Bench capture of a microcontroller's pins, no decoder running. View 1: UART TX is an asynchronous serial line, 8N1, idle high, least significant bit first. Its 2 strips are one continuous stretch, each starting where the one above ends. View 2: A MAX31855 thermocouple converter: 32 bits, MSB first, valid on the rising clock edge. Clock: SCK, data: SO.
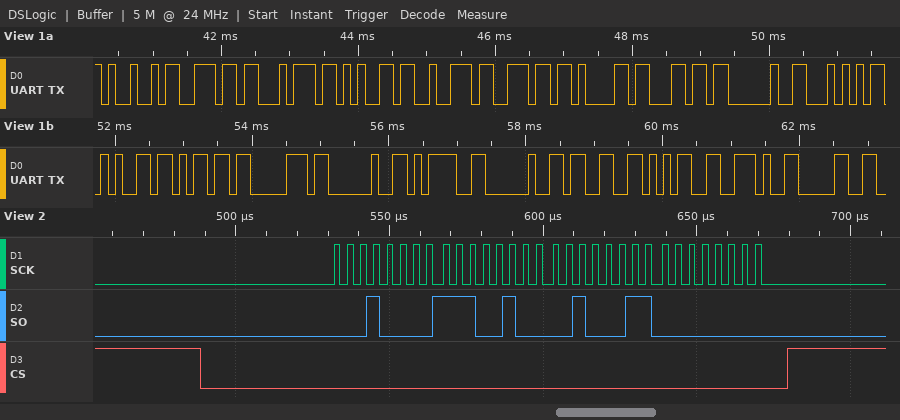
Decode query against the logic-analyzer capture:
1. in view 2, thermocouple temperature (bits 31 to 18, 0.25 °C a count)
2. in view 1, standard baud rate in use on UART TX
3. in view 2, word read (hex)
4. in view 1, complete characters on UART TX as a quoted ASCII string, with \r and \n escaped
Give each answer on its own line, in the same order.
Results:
270.25 °C
9600 baud
0x10E42300
"Internal Temp = 35.0"
